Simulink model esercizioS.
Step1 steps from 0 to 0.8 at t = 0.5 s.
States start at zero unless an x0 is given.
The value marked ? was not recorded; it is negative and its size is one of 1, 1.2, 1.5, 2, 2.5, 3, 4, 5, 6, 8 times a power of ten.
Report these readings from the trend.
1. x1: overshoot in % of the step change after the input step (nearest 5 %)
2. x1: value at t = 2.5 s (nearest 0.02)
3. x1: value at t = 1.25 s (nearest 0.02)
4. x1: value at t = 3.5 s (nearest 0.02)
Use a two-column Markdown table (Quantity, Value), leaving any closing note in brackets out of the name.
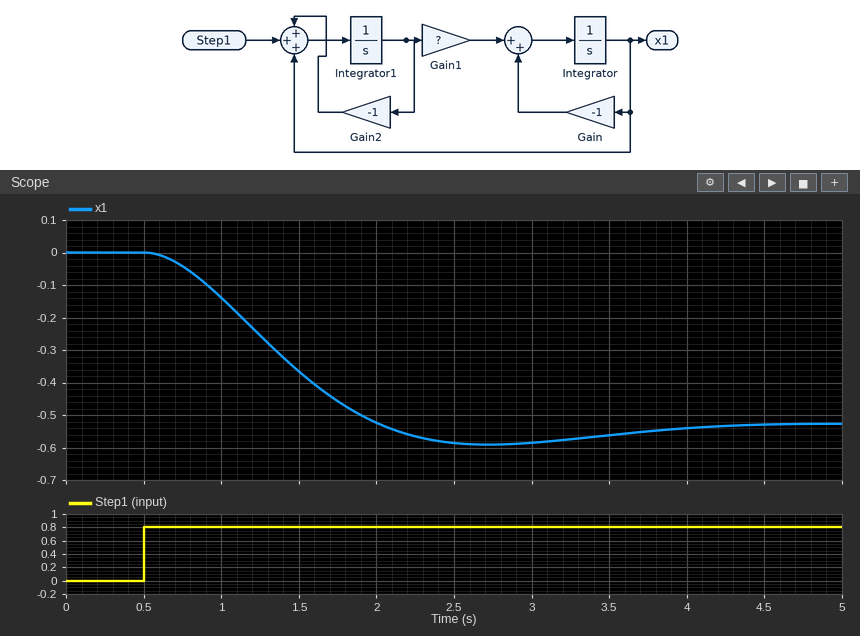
| Quantity | Value |
|---|---|
| x1: overshoot in % of the step change after the input step | 10 % |
| x1: value at t = 2.5 s | -0.58 |
| x1: value at t = 1.25 s | -0.26 |
| x1: value at t = 3.5 s | -0.56 |
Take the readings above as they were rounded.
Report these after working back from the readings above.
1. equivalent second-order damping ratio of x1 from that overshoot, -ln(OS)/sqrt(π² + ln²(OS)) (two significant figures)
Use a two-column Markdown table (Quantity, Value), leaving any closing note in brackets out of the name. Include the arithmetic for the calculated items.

| Quantity | Value |
|---|---|
| equivalent second-order damping ratio of x1 from that overshoot, -ln(OS)/sqrt(π² + ln²(OS)) | ln(0.1) = -2.303; 2.303 / sqrt(9.870 + 5.302) = 0.59 |
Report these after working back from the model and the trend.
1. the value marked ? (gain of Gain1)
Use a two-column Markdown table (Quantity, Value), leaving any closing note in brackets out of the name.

| Quantity | Value |
|---|---|
| the value marked ? | -2 |
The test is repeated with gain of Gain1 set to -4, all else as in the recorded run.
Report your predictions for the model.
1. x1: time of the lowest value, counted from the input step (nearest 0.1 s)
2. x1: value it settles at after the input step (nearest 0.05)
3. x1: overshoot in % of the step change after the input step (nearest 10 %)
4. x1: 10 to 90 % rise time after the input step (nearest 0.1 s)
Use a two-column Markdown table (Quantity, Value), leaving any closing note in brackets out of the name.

| Quantity | Value |
|---|---|
| x1: time of the lowest value, counted from the input step | 1.6 s |
| x1: value it settles at after the input step | -0.65 |
| x1: overshoot in % of the step change after the input step | 20 % |
| x1: 10 to 90 % rise time after the input step | 0.7 s |
